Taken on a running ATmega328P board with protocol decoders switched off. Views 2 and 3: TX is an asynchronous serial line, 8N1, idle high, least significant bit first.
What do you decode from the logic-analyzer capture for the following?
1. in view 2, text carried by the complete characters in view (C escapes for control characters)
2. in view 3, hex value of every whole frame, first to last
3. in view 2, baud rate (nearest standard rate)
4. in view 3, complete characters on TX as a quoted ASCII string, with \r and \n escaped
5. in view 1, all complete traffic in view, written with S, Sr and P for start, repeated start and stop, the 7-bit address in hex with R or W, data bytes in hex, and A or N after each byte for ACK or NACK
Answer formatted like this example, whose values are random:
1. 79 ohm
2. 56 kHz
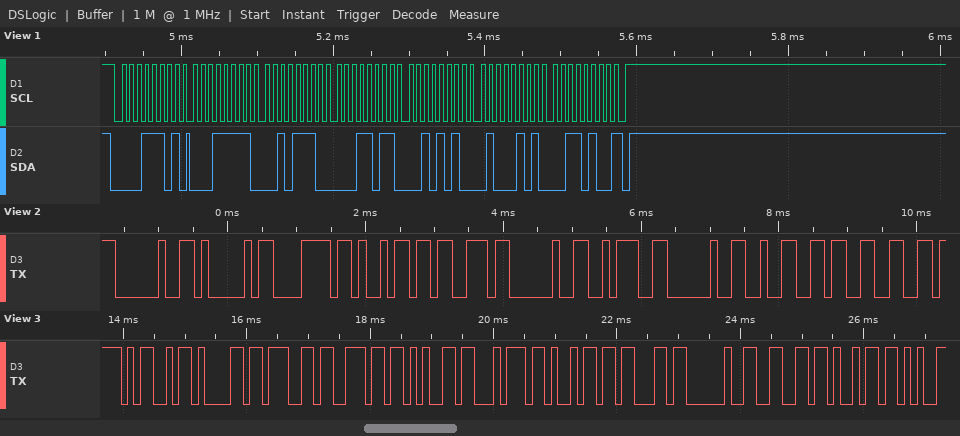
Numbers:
1. " Axis : 23"
2. 0x4D 0x61 0x67 0x6E 0x65 0x74 0x69 0x63 0x20 0x66 0x69
3. 9600 baud
4. "Magnetic fi"
5. S 0ER A 1F A 2E A 1B A 2A A 45 A 34 N P
